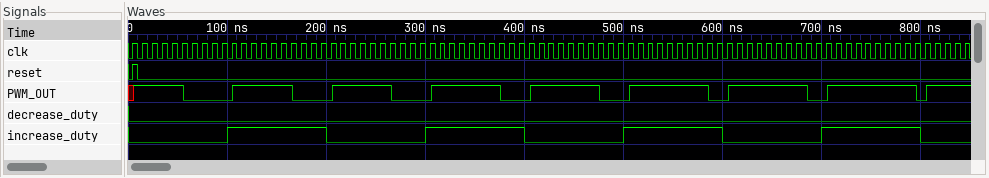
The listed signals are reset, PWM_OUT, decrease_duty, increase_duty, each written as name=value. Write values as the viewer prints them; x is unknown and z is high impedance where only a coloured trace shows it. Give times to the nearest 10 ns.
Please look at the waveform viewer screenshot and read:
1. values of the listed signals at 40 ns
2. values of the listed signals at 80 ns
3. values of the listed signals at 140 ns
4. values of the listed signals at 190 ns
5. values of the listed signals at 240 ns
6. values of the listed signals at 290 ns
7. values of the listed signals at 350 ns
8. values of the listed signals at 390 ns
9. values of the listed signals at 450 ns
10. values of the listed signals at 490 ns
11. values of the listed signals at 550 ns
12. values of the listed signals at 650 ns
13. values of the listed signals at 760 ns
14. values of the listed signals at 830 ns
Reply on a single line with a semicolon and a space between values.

reset=0, PWM_OUT=1, decrease_duty=0, increase_duty=0; reset=0, PWM_OUT=0, decrease_duty=0, increase_duty=0; reset=0, PWM_OUT=1, decrease_duty=0, increase_duty=1; reset=0, PWM_OUT=0, decrease_duty=0, increase_duty=1; reset=0, PWM_OUT=1, decrease_duty=0, increase_duty=0; reset=0, PWM_OUT=0, decrease_duty=0, increase_duty=0; reset=0, PWM_OUT=1, decrease_duty=0, increase_duty=1; reset=0, PWM_OUT=0, decrease_duty=0, increase_duty=1; reset=0, PWM_OUT=1, decrease_duty=0, increase_duty=0; reset=0, PWM_OUT=0, decrease_duty=0, increase_duty=0; reset=0, PWM_OUT=1, decrease_duty=0, increase_duty=1; reset=0, PWM_OUT=1, decrease_duty=0, increase_duty=0; reset=0, PWM_OUT=1, decrease_duty=0, increase_duty=1; reset=0, PWM_OUT=1, decrease_duty=0, increase_duty=0
